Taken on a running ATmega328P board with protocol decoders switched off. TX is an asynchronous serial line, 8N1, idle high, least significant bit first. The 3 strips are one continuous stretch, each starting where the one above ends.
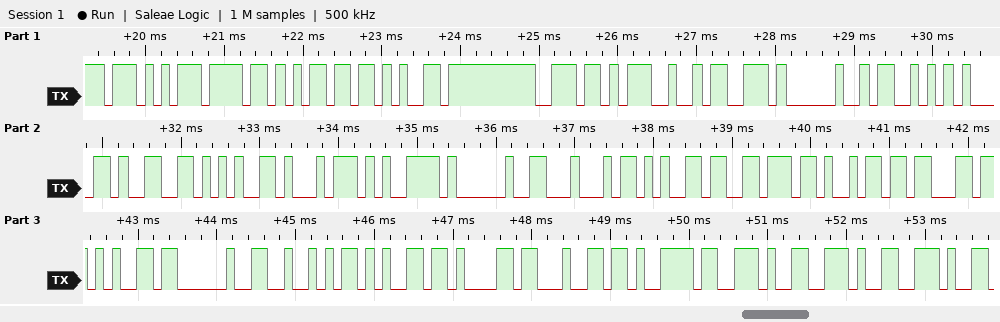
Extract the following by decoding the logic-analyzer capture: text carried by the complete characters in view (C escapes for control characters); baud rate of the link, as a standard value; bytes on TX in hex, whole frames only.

"Women's Safety Device Ready..."
9600 baud
57 6F 6D 65 6E 27 73 20 53 61 66 65 74 79 20 44 65 76 69 63 65 20 52 65 61 64 79 2E 2E 2E
